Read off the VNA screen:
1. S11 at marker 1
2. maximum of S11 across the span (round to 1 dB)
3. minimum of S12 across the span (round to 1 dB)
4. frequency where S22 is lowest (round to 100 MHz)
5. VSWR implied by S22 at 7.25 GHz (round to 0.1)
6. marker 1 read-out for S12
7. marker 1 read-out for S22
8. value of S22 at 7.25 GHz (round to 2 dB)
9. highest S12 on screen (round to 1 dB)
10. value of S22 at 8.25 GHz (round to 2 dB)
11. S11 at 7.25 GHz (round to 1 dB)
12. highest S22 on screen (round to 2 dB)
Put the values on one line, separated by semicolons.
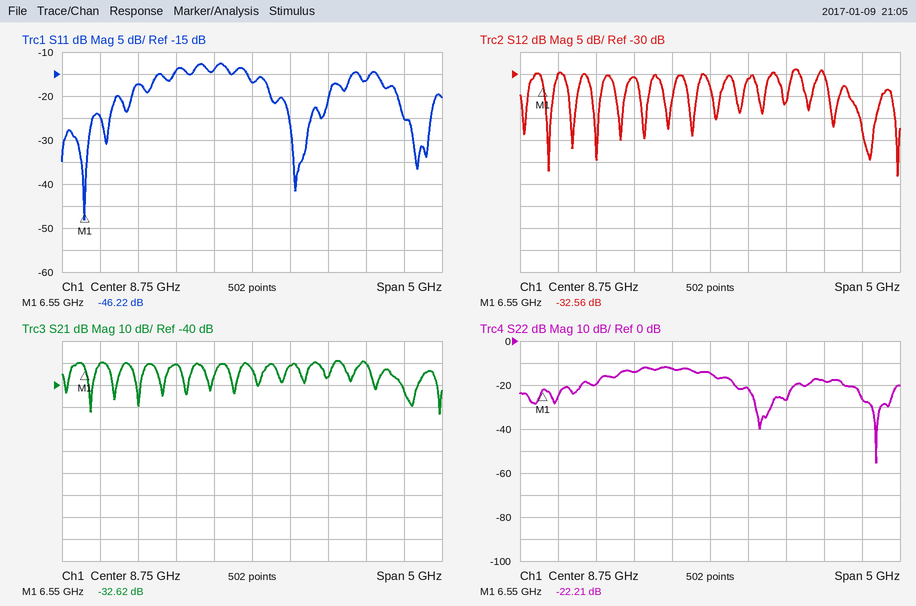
-46.22 dB; -13 dB; -53 dB; 10.9 GHz; 1.2; -32.56 dB; -22.21 dB; -20 dB; -29 dB; -12 dB; -17 dB; -12 dB
